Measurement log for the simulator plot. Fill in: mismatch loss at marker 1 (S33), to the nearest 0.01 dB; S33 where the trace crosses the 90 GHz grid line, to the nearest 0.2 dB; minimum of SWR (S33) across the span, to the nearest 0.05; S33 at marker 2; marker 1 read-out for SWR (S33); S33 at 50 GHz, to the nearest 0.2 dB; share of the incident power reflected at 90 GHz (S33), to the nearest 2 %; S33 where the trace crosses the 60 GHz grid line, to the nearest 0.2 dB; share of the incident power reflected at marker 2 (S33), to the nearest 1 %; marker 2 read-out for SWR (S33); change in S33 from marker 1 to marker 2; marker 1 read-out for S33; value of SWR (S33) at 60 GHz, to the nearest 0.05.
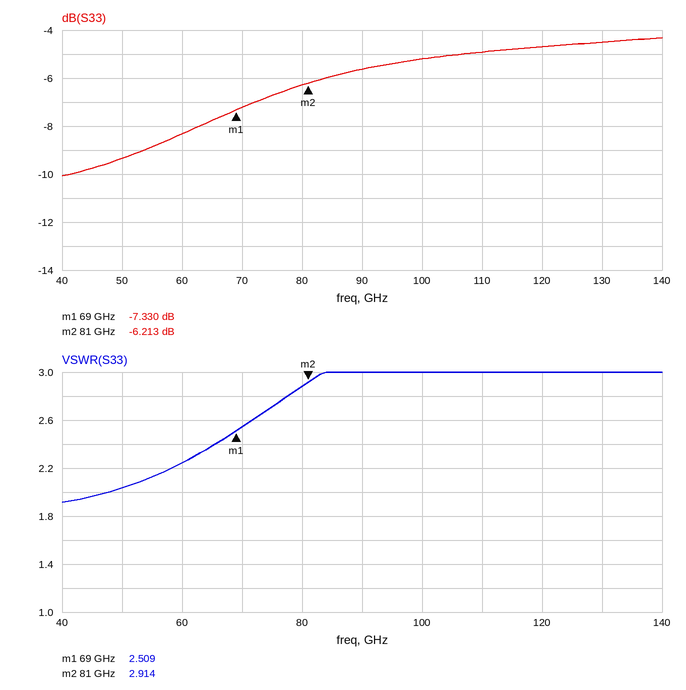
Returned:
0.89 dB
-5.6 dB
1.90
-6.213 dB
2.509
-9.4 dB
28 %
-8.4 dB
24 %
2.914
1.117 dB
-7.330 dB
2.25
